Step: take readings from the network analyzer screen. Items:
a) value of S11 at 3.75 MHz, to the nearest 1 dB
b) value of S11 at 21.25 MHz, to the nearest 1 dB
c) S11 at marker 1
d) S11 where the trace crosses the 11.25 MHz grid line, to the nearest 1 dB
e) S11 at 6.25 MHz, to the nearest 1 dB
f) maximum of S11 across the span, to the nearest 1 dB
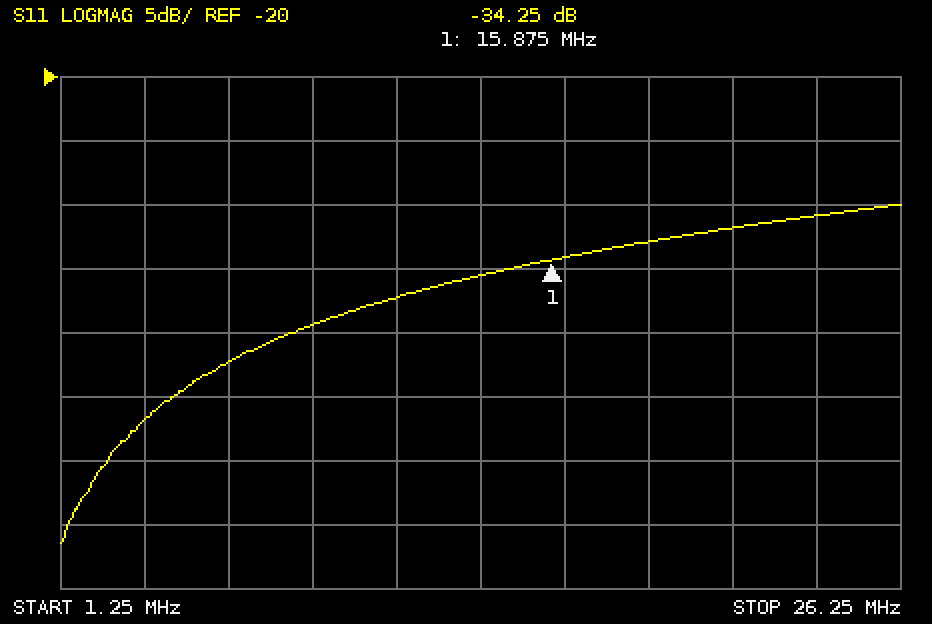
-47 dB
-32 dB
-34.25 dB
-37 dB
-42 dB
-30 dB
